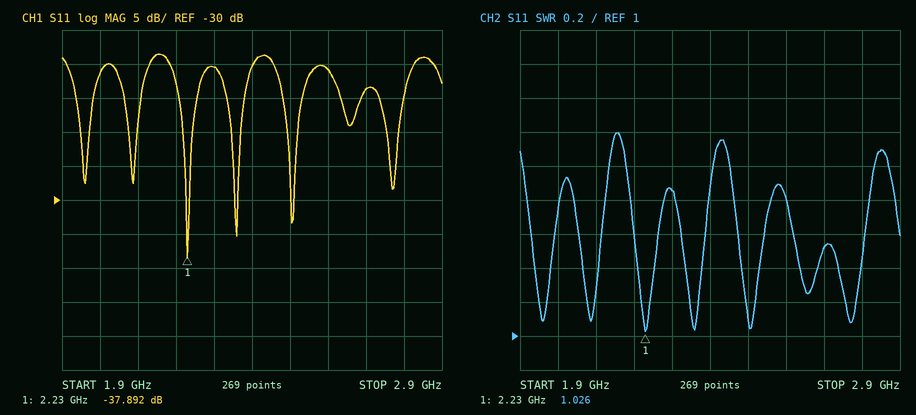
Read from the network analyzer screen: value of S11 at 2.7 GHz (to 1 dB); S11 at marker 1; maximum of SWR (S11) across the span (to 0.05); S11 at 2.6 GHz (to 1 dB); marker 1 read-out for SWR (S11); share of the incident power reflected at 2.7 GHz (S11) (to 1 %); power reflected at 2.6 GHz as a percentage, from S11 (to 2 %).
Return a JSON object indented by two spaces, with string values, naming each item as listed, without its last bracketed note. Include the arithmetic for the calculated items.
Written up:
{
  "value of S11 at 2.7 GHz": "-14 dB",
  "S11 at marker 1": "-37.892 dB",
  "maximum of SWR (S11) across the span": "2.20",
  "S11 at 2.6 GHz": "-11 dB",
  "marker 1 read-out for SWR": "1.026",
  "share of the incident power reflected at 2.7 GHz (S11)": "10^(-14/10) ≈ 4 %",
  "power reflected at 2.6 GHz as a percentage, from S11": "10^(-11/10) ≈ 8 %"
}
